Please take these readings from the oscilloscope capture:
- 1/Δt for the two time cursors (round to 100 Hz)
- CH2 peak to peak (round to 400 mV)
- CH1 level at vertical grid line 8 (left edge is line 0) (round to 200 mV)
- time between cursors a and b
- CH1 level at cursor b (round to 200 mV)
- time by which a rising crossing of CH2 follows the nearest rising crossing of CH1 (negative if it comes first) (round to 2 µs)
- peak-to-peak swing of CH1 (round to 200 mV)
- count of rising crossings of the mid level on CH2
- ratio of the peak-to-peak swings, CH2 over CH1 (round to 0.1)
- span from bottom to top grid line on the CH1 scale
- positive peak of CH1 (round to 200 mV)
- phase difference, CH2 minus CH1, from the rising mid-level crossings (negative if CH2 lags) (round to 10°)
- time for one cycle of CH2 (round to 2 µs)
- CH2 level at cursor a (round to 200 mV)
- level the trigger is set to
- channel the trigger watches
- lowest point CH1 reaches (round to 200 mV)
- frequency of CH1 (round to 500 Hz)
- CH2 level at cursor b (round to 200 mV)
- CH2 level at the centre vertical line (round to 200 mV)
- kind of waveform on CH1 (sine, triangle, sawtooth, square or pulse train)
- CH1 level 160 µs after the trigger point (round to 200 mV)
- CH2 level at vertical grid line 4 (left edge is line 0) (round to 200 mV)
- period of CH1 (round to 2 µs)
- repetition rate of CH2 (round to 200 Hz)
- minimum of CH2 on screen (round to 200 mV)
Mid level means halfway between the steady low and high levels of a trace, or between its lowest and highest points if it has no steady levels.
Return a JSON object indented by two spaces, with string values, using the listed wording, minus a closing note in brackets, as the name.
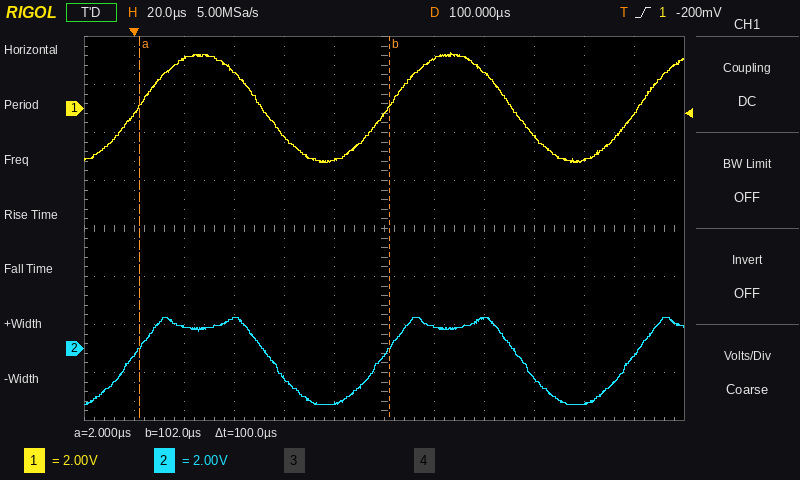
{
  "1/Δt for the two time cursors": "10.0 kHz",
  "CH2 peak to peak": "3.6 V",
  "CH1 level at vertical grid line 8 (left edge is line 0)": "1.4 V",
  "time between cursors a and b": "100 µs",
  "CH1 level at cursor b": "0.0 V",
  "time by which a rising crossing of CH2 follows the nearest rising crossing of CH1 (negative if it comes first)": "-4 µs",
  "peak-to-peak swing of CH1": "4.6 V",
  "count of rising crossings of the mid level on CH2": "3",
  "ratio of the peak-to-peak swings, CH2 over CH1": "0.8",
  "span from bottom to top grid line on the CH1 scale": "16 V",
  "positive peak of CH1": "2.4 V",
  "phase difference, CH2 minus CH1, from the rising mid-level crossings (negative if CH2 lags)": "+10°",
  "time for one cycle of CH2": "100 µs",
  "CH2 level at cursor a": "0.0 V",
  "level the trigger is set to": "-200 mV",
  "channel the trigger watches": "CH1",
  "lowest point CH1 reaches": "-2.2 V",
  "frequency of CH1": "10.0 kHz",
  "CH2 level at cursor b": "0.0 V",
  "CH2 level at the centre vertical line": "-200 mV",
  "kind of waveform on CH1": "sine",
  "CH1 level 160 µs after the trigger point": "-1.2 V",
  "CH2 level at vertical grid line 4 (left edge is line 0)": "-1.2 V",
  "period of CH1": "100 µs",
  "repetition rate of CH2": "10.0 kHz",
  "minimum of CH2 on screen": "-2.4 V"
}
